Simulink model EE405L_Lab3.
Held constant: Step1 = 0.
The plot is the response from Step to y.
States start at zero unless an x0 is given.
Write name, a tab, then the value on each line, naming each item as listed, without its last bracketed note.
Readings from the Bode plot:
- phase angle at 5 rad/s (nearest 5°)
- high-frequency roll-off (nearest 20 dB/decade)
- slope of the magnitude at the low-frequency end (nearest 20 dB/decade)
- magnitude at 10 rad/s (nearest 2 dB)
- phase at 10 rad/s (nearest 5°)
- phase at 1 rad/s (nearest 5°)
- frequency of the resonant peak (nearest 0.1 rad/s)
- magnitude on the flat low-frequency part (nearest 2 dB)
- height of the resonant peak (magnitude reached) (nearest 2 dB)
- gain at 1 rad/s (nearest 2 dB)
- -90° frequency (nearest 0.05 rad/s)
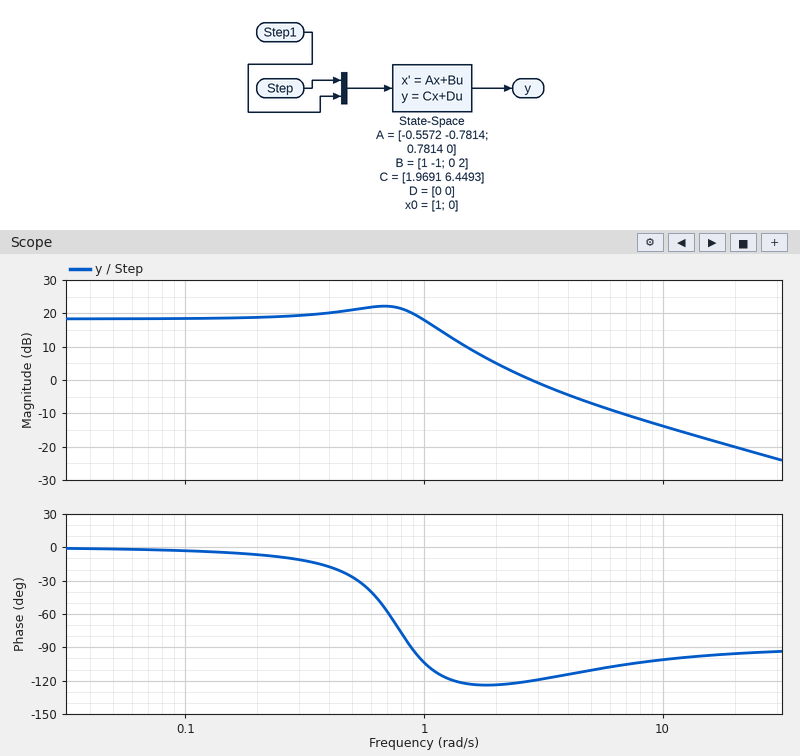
phase angle at 5 rad/s	-110°
high-frequency roll-off	-20 dB/decade
slope of the magnitude at the low-frequency end	0 dB/decade
magnitude at 10 rad/s	-14 dB
phase at 10 rad/s	-100°
phase at 1 rad/s	-105°
frequency of the resonant peak	0.7 rad/s
magnitude on the flat low-frequency part	18 dB
height of the resonant peak (magnitude reached)	22 dB
gain at 1 rad/s	18 dB
-90° frequency	0.90 rad/s
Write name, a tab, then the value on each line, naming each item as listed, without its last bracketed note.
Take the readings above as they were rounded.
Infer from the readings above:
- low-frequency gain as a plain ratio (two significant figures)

low-frequency gain as a plain ratio	7.9
